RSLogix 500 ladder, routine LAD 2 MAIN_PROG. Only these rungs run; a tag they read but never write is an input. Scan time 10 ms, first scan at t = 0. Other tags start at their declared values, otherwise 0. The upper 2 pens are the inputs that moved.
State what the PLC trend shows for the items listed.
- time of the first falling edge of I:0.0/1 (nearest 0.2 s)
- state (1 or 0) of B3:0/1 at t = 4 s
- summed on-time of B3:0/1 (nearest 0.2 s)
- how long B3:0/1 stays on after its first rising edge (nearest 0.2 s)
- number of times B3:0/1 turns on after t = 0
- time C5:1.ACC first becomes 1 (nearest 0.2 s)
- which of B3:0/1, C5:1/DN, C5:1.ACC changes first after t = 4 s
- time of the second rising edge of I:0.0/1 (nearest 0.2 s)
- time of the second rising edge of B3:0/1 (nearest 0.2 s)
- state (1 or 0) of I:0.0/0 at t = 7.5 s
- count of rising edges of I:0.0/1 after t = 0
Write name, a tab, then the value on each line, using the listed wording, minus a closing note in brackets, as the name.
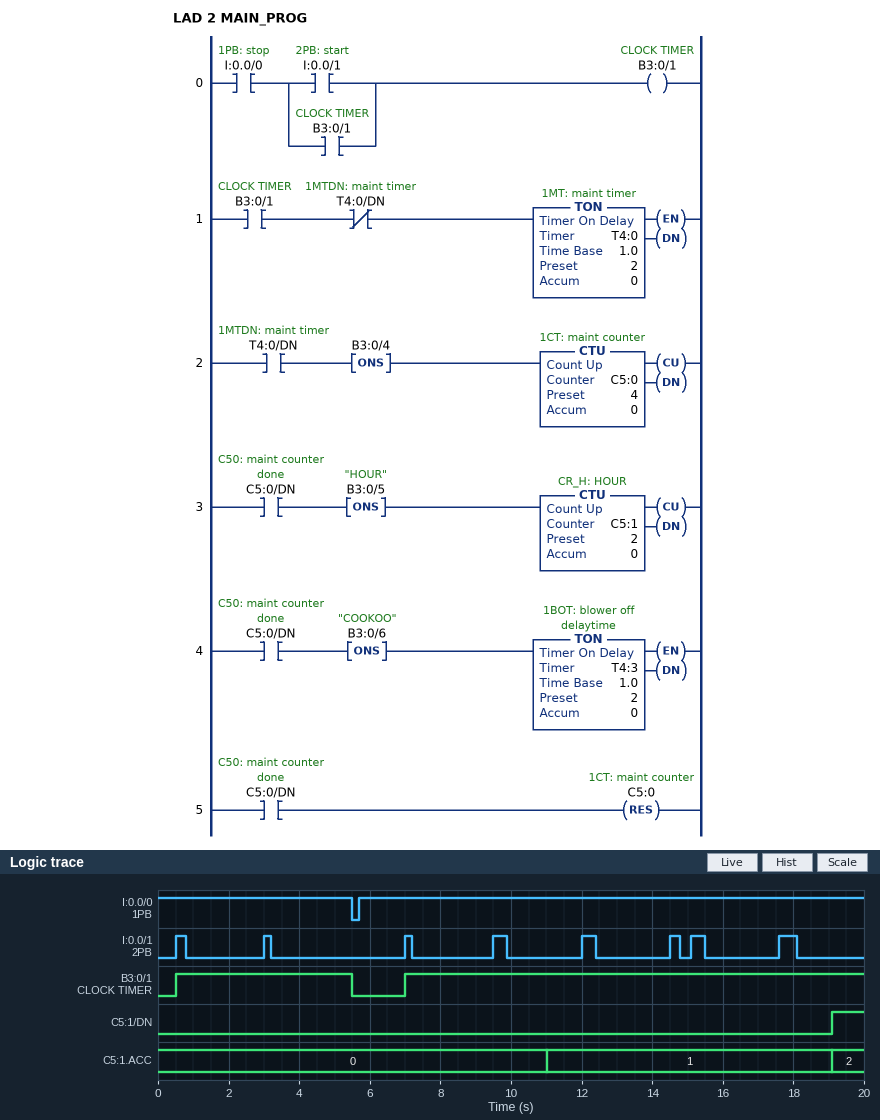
time of the first falling edge of I:0.0/1	0.8 s
state (1 or 0) of B3:0/1 at t = 4 s	1
summed on-time of B3:0/1	18.0 s
how long B3:0/1 stays on after its first rising edge	5.0 s
number of times B3:0/1 turns on after t = 0	2
time C5:1.ACC first becomes 1	11.0 s
which of B3:0/1, C5:1/DN, C5:1.ACC changes first after t = 4 s	B3:0/1
time of the second rising edge of I:0.0/1	3.0 s
time of the second rising edge of B3:0/1	7.0 s
state (1 or 0) of I:0.0/0 at t = 7.5 s	1
count of rising edges of I:0.0/1 after t = 0	8
